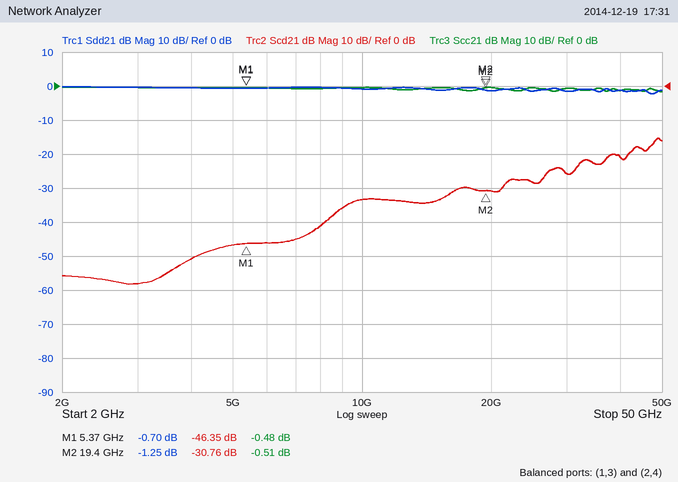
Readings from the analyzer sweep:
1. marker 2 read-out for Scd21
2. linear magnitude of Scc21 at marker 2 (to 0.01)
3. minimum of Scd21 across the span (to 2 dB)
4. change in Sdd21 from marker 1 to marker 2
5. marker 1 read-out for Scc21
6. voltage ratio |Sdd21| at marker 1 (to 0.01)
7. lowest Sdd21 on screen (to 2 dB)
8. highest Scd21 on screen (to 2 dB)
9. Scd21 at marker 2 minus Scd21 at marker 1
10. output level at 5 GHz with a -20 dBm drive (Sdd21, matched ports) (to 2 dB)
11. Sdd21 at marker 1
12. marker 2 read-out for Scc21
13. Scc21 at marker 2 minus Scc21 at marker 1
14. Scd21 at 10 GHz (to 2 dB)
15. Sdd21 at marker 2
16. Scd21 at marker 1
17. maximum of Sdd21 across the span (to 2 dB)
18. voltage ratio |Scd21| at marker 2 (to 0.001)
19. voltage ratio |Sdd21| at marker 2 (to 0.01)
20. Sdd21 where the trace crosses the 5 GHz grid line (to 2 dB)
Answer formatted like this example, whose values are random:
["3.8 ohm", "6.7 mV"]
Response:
["-30.76 dB", "0.94", "-58 dB", "-0.55 dB", "-0.48 dB", "0.92", "-2 dB", "-16 dB", "15.59 dB", "-20 dBm", "-0.70 dB", "-0.51 dB", "-0.03 dB", "-34 dB", "-1.25 dB", "-46.35 dB", "0 dB", "0.029", "0.87", "0 dB"]
